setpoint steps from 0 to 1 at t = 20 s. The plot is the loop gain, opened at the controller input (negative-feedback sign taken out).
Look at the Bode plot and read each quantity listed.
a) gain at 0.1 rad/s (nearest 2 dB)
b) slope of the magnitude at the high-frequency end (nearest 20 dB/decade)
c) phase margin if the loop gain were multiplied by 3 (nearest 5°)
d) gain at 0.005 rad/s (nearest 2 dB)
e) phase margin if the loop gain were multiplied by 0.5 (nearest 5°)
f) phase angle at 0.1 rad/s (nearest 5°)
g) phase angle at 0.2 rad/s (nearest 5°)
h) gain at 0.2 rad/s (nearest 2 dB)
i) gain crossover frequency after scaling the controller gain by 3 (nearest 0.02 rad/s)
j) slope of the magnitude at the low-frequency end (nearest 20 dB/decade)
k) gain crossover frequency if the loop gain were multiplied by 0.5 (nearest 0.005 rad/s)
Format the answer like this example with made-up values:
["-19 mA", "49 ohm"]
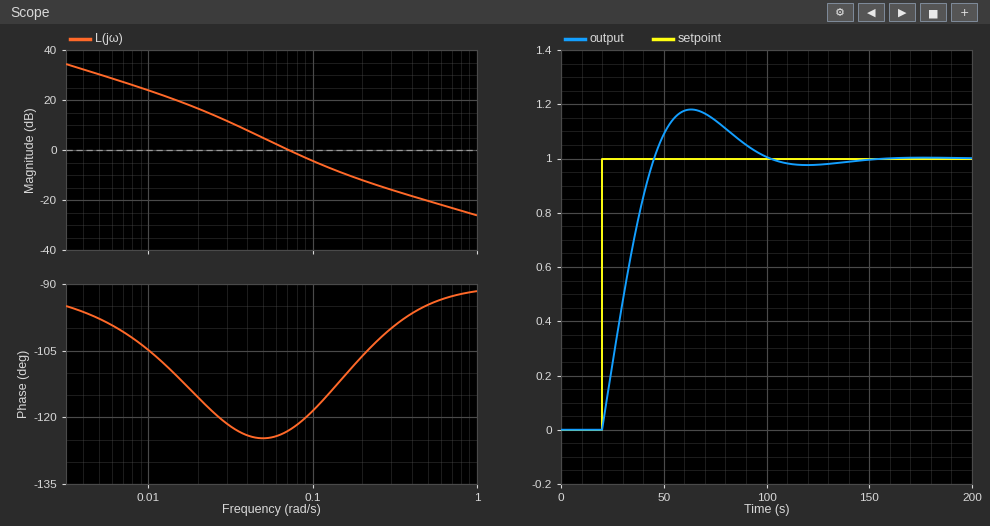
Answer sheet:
["-4 dB", "-20 dB/decade", "70°", "30 dB", "55°", "-120°", "-105°", "-12 dB", "0.16 rad/s", "-20 dB/decade", "0.045 rad/s"]
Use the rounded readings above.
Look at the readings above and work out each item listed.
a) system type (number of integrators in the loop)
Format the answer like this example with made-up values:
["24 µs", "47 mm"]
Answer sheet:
["1"]
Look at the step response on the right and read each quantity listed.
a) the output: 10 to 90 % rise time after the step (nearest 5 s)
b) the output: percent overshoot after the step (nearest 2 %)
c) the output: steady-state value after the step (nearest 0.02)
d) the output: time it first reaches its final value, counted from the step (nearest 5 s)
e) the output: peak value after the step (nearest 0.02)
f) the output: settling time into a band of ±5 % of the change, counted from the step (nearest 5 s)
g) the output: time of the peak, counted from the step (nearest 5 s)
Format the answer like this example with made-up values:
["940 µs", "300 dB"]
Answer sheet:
["20 s", "18 %", "1.00", "25 s", "1.18", "70 s", "45 s"]
